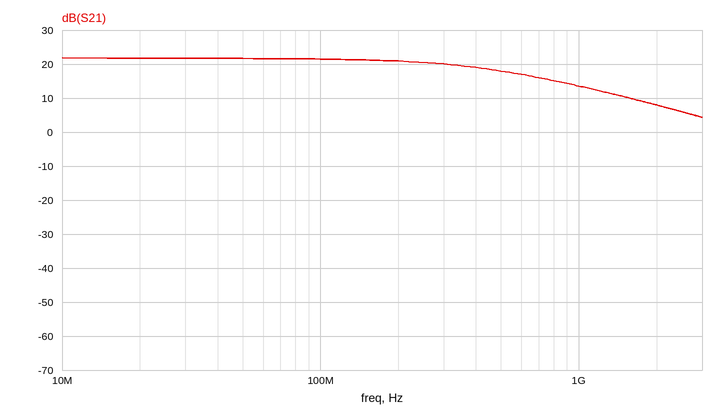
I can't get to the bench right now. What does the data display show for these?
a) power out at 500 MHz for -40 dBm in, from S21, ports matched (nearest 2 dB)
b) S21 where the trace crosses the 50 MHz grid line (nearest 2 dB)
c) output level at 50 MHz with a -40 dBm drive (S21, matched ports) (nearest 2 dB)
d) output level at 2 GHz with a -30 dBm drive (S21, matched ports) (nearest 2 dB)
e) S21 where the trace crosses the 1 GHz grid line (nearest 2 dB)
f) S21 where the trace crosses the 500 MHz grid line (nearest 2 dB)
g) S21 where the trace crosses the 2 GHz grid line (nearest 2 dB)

-22 dBm
22 dB
-18 dBm
-22 dBm
14 dB
18 dB
8 dB
